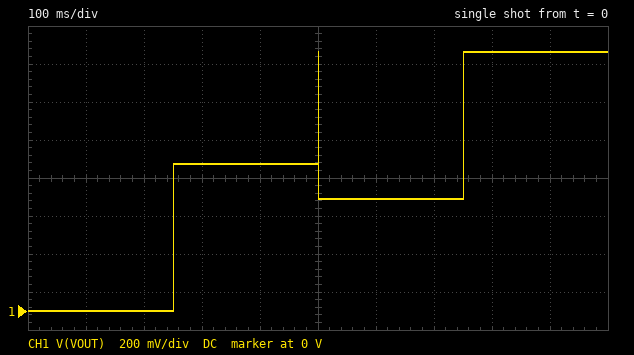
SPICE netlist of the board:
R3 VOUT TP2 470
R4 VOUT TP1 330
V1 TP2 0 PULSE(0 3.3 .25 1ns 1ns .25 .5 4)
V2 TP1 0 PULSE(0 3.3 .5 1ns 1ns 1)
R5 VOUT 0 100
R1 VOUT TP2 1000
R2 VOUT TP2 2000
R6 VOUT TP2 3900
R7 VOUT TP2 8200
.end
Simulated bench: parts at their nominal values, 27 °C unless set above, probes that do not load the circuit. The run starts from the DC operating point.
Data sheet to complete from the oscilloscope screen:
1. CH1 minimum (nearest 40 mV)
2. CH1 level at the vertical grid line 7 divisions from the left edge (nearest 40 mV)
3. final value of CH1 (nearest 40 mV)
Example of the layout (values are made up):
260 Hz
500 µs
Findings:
0 V
600 mV
1.36 V
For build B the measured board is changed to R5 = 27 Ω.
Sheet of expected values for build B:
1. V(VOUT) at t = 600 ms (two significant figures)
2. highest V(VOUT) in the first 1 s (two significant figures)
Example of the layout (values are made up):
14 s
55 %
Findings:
230 mV
530 mV
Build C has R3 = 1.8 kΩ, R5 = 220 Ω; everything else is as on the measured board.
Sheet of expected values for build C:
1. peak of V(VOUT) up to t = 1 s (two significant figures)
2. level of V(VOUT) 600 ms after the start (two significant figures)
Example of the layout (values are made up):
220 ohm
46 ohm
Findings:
1.8 V
1.0 V
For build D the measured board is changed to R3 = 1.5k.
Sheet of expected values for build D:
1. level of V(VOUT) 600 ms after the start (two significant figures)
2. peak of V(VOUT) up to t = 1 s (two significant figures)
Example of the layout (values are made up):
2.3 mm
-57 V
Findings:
640 mV
1.2 V
